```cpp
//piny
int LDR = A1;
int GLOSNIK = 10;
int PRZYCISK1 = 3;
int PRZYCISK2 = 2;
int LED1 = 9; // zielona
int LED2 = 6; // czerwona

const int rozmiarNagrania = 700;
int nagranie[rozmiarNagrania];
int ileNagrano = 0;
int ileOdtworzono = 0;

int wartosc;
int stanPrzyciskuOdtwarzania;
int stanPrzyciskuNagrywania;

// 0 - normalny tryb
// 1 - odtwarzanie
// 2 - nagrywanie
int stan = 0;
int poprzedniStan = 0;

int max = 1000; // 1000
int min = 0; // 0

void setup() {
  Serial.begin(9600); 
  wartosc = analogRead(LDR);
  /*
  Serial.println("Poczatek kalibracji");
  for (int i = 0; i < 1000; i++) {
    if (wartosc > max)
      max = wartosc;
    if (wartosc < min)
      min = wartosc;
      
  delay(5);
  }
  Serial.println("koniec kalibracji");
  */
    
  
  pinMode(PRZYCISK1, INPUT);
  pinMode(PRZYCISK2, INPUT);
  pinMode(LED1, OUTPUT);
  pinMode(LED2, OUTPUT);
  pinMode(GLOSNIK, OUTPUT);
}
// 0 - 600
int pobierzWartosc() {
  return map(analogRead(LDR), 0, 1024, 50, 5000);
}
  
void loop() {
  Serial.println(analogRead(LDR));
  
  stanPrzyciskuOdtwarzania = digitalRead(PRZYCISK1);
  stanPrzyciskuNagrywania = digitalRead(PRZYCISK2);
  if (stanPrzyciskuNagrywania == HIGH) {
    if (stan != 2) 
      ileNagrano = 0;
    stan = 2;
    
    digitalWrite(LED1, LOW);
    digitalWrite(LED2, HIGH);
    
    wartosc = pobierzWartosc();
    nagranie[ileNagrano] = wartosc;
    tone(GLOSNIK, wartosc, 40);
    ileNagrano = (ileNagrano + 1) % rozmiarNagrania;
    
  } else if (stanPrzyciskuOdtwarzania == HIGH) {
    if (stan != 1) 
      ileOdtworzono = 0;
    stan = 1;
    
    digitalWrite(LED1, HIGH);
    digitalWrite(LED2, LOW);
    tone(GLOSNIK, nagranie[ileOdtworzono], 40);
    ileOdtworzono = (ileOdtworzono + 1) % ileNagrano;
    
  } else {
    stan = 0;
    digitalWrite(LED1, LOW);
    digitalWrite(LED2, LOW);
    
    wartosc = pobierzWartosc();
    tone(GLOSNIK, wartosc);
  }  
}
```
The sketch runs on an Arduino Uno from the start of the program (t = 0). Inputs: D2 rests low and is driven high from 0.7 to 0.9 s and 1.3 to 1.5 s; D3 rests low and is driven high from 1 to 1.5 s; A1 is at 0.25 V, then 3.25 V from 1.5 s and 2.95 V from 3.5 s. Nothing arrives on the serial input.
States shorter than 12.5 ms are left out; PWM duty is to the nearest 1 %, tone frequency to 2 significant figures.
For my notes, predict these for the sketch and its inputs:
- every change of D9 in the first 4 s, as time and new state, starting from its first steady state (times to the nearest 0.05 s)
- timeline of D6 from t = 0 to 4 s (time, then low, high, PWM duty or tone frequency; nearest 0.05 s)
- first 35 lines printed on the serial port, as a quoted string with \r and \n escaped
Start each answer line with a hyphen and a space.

- 0 s low; 1 s high; 1.3 s low
- 0 s low; 0.7 s high; 0.9 s low; 1.3 s high; 1.5 s low
- "51\r\n51\r\n51\r\n51\r\n51\r\n51\r\n51\r\n51\r\n51\r\n51\r\n51\r\n51\r\n51\r\n51\r\n51\r\n51\r\n51\r\n51\r\n51\r\n51\r\n51\r\n51\r\n51\r\n51\r\n51\r\n51\r\n51\r\n51\r\n51\r\n51\r\n51\r\n51\r\n51\r\n51\r\n51\r\n"
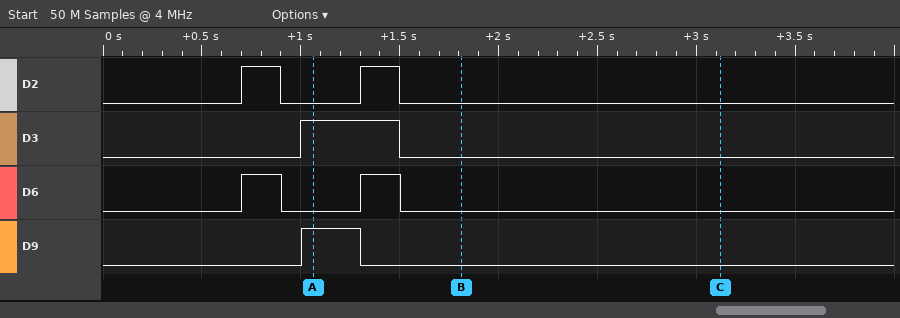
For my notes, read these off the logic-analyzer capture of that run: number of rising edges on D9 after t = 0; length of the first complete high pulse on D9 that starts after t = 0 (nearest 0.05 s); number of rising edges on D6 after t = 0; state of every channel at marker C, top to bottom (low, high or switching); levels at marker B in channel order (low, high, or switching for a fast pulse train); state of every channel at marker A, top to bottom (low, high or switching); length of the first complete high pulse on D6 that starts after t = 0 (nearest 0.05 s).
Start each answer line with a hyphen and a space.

- 1
- 0.30 s
- 2
- D2 low, D3 low, D6 low, D9 low
- D2 low, D3 low, D6 low, D9 low
- D2 low, D3 high, D6 low, D9 high
- 0.20 s
